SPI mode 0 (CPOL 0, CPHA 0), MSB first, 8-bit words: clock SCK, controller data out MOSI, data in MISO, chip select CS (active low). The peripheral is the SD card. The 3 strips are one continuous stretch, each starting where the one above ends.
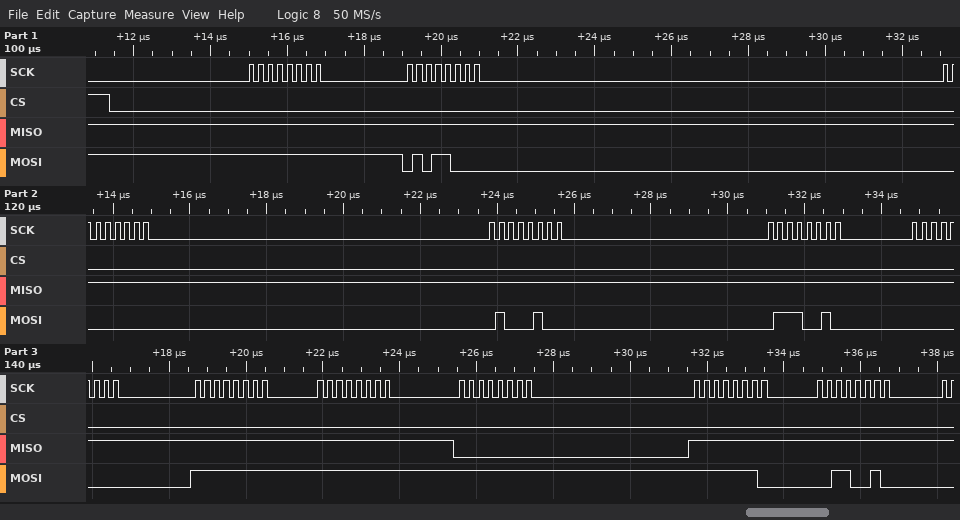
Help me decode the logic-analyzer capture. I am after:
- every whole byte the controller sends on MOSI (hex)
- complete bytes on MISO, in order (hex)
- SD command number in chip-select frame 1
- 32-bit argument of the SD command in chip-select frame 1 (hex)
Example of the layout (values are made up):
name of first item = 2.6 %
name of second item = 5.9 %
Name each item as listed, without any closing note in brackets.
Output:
every whole byte the controller sends on MOSI = FF 58 00 44 72 00 FF FF FF FE 32
complete bytes on MISO, in order = FF FF FF FF FF FF FF FF 00 FF FF
SD command number in chip-select frame 1 = CMD24
32-bit argument of the SD command in chip-select frame 1 = 0x00447200
